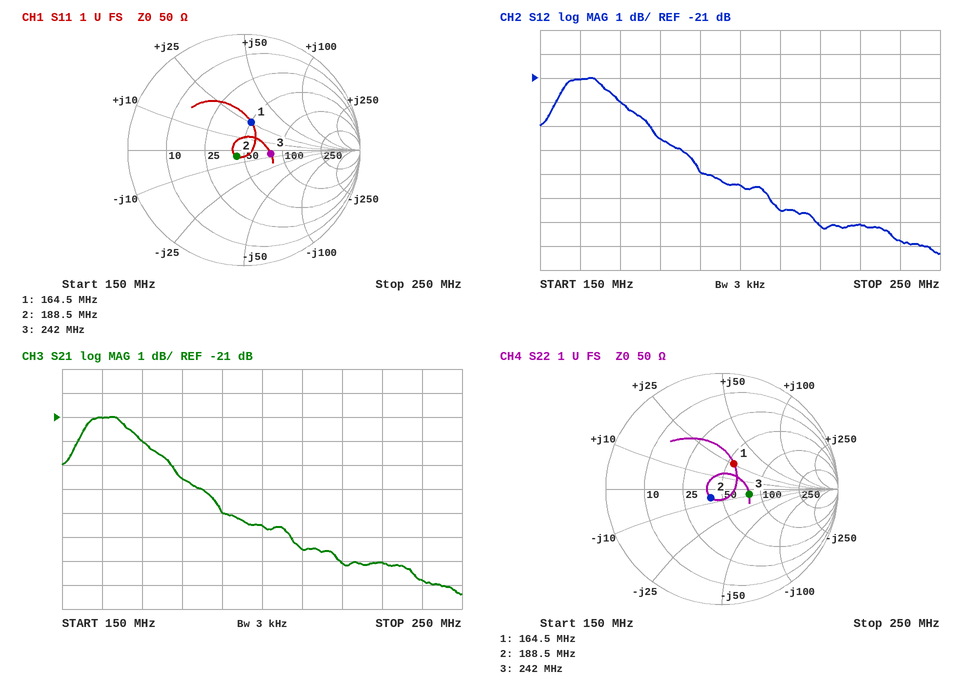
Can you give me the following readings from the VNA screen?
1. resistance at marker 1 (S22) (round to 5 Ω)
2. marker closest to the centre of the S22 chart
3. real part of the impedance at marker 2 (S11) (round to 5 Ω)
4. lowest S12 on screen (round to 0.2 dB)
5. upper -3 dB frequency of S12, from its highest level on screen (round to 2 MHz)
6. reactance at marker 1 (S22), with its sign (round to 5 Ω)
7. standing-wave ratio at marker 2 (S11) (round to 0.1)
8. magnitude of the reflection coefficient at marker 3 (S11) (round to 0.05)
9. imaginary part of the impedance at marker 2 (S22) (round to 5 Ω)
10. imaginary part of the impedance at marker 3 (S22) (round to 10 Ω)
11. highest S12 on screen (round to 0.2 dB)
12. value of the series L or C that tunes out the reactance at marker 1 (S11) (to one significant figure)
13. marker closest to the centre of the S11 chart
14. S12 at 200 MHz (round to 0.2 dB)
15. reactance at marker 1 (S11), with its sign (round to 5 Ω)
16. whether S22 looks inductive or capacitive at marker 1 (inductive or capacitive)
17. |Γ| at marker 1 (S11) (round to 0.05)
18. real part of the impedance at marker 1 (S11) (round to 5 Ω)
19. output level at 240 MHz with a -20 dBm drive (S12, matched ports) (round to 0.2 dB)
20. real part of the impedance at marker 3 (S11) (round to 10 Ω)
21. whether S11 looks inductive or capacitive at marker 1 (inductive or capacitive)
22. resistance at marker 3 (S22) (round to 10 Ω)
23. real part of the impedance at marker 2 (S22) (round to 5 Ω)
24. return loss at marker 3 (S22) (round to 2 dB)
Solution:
55 Ω
marker 2
45 Ω
-28.4 dB
186 MHz
+25 Ω
1.2
0.25
-5 Ω
-10 Ω
-21.0 dB
40 pF
marker 2
-25.4 dB
+25 Ω
inductive
0.25
50 Ω
-47.8 dBm
80 Ω
inductive
80 Ω
40 Ω
12 dB
